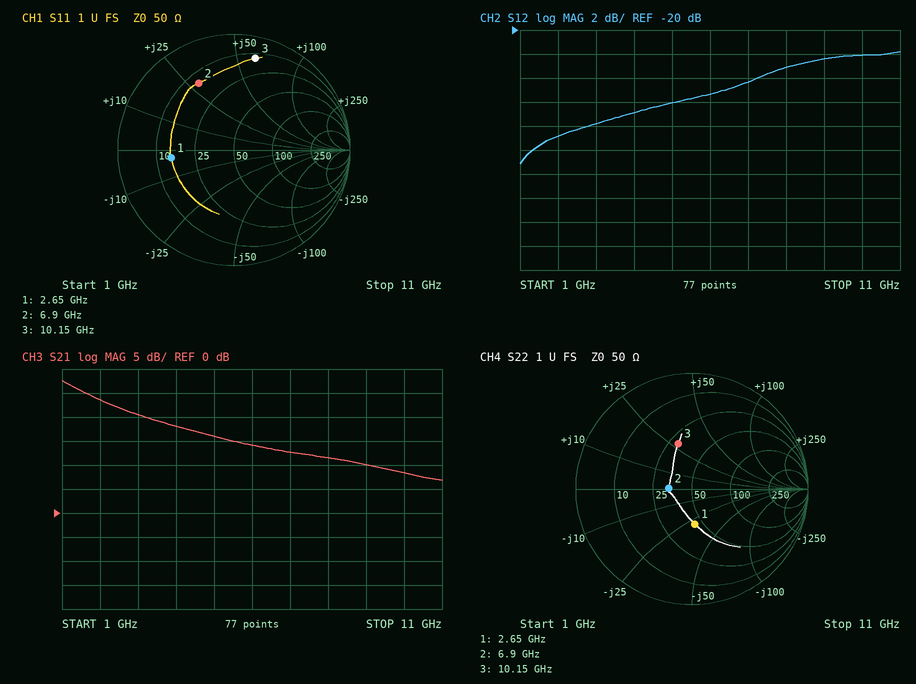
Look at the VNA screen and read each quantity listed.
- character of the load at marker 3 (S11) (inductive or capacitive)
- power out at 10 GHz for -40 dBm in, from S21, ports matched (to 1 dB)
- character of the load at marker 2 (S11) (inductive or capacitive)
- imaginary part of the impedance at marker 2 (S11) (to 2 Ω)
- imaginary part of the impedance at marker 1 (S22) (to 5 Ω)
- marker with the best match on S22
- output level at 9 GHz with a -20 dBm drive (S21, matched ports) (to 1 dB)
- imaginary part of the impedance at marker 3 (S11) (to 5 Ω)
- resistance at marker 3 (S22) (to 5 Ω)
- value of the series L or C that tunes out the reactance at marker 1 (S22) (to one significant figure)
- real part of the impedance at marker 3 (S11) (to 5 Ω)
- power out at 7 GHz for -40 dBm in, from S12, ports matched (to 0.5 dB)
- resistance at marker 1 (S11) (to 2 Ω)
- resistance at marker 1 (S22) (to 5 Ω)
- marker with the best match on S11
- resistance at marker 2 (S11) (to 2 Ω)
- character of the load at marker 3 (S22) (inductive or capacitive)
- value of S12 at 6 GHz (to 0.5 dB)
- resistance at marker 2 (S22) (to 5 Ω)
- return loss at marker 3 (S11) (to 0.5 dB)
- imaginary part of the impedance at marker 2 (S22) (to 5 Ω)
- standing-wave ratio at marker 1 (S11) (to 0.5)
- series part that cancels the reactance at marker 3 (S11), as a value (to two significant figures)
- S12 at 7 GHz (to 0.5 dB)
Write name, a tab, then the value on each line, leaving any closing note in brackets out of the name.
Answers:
character of the load at marker 3 (S11)	inductive
power out at 10 GHz for -40 dBm in, from S21, ports matched	-32 dBm
character of the load at marker 2 (S11)	inductive
imaginary part of the impedance at marker 2 (S11)	+28 Ω
imaginary part of the impedance at marker 1 (S22)	-30 Ω
marker with the best match on S22	marker 2
output level at 9 GHz with a -20 dBm drive (S21, matched ports)	-10 dBm
imaginary part of the impedance at marker 3 (S11)	+60 Ω
resistance at marker 3 (S22)	30 Ω
value of the series L or C that tunes out the reactance at marker 1 (S22)	2 nH
real part of the impedance at marker 3 (S11)	15 Ω
power out at 7 GHz for -40 dBm in, from S12, ports matched	-64.5 dBm
resistance at marker 1 (S11)	14 Ω
resistance at marker 1 (S22)	45 Ω
marker with the best match on S11	marker 1
resistance at marker 2 (S11)	14 Ω
character of the load at marker 3 (S22)	inductive
value of S12 at 6 GHz	-25.5 dB
resistance at marker 2 (S22)	35 Ω
return loss at marker 3 (S11)	2.0 dB
imaginary part of the impedance at marker 2 (S22)	0 Ω
standing-wave ratio at marker 1 (S11)	3.5
series part that cancels the reactance at marker 3 (S11), as a value	260 fF
S12 at 7 GHz	-24.5 dB
